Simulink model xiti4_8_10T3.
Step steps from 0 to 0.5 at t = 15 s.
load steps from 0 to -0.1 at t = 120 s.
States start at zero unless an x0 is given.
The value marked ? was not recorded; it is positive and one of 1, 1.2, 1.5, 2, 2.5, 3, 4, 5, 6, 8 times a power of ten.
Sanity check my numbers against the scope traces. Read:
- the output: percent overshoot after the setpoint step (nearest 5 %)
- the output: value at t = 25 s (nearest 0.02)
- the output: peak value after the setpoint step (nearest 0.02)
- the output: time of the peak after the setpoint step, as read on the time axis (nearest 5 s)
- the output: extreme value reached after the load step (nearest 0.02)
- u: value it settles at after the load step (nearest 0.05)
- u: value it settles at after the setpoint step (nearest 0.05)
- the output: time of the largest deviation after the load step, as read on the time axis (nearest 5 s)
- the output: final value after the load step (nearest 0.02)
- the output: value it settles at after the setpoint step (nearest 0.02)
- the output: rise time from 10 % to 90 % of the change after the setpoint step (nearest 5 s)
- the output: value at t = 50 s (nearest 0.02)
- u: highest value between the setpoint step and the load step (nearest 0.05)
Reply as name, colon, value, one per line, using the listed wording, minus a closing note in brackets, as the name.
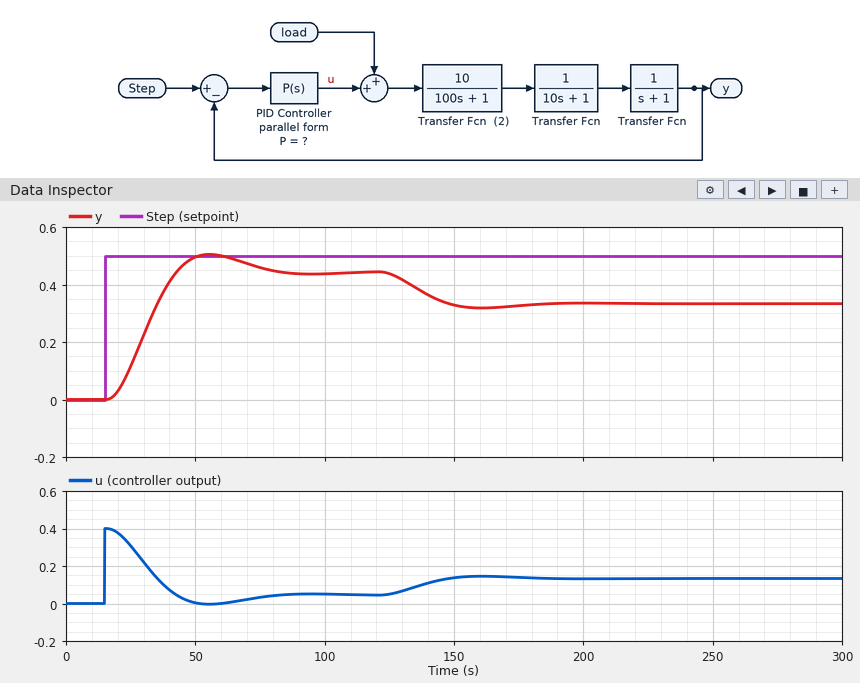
the output: percent overshoot after the setpoint step: 15 %
the output: value at t = 25 s: 0.12
the output: peak value after the setpoint step: 0.50
the output: time of the peak after the setpoint step, as read on the time axis: 55 s
the output: extreme value reached after the load step: 0.32
u: value it settles at after the load step: 0.15
u: value it settles at after the setpoint step: 0.05
the output: time of the largest deviation after the load step, as read on the time axis: 160 s
the output: final value after the load step: 0.34
the output: value it settles at after the setpoint step: 0.44
the output: rise time from 10 % to 90 % of the change after the setpoint step: 20 s
the output: value at t = 50 s: 0.50
u: highest value between the setpoint step and the load step: 0.40
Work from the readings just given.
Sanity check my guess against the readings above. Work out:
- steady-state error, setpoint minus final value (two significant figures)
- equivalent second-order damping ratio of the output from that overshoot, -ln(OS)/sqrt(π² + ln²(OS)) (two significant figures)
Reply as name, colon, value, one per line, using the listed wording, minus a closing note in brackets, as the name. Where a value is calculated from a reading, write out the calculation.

steady-state error, setpoint minus final value: 0.5 - 0.44 = 0.060
equivalent second-order damping ratio of the output from that overshoot, -ln(OS)/sqrt(π² + ln²(OS)): ln(0.15) = -1.897; 1.897 / sqrt(9.870 + 3.599) = 0.52
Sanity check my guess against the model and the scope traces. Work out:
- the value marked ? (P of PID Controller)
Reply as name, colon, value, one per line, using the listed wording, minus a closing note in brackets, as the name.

the value marked ?: 0.8
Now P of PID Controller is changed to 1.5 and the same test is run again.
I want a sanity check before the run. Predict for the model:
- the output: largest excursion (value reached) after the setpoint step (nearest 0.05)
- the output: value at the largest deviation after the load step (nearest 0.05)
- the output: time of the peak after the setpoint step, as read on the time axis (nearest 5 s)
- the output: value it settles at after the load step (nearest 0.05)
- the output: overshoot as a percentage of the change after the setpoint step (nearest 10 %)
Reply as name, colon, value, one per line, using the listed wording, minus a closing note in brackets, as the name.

the output: largest excursion (value reached) after the setpoint step: 0.60
the output: value at the largest deviation after the load step: 0.40
the output: time of the peak after the setpoint step, as read on the time axis: 45 s
the output: value it settles at after the load step: 0.40
the output: overshoot as a percentage of the change after the setpoint step: 30 %
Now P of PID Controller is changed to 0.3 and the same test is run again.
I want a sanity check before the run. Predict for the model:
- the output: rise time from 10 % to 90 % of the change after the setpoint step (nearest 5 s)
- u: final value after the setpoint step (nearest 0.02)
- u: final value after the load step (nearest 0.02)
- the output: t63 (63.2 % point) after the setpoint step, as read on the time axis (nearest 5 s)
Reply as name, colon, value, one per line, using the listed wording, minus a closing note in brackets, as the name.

the output: rise time from 10 % to 90 % of the change after the setpoint step: 40 s
u: final value after the setpoint step: 0.04
u: final value after the load step: 0.12
the output: t63 (63.2 % point) after the setpoint step, as read on the time axis: 45 s
